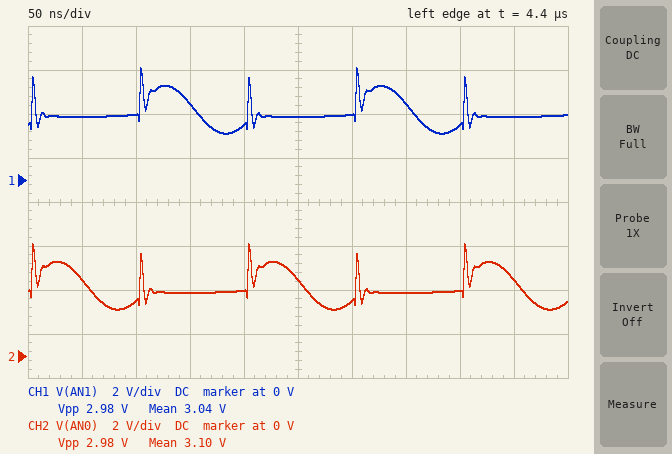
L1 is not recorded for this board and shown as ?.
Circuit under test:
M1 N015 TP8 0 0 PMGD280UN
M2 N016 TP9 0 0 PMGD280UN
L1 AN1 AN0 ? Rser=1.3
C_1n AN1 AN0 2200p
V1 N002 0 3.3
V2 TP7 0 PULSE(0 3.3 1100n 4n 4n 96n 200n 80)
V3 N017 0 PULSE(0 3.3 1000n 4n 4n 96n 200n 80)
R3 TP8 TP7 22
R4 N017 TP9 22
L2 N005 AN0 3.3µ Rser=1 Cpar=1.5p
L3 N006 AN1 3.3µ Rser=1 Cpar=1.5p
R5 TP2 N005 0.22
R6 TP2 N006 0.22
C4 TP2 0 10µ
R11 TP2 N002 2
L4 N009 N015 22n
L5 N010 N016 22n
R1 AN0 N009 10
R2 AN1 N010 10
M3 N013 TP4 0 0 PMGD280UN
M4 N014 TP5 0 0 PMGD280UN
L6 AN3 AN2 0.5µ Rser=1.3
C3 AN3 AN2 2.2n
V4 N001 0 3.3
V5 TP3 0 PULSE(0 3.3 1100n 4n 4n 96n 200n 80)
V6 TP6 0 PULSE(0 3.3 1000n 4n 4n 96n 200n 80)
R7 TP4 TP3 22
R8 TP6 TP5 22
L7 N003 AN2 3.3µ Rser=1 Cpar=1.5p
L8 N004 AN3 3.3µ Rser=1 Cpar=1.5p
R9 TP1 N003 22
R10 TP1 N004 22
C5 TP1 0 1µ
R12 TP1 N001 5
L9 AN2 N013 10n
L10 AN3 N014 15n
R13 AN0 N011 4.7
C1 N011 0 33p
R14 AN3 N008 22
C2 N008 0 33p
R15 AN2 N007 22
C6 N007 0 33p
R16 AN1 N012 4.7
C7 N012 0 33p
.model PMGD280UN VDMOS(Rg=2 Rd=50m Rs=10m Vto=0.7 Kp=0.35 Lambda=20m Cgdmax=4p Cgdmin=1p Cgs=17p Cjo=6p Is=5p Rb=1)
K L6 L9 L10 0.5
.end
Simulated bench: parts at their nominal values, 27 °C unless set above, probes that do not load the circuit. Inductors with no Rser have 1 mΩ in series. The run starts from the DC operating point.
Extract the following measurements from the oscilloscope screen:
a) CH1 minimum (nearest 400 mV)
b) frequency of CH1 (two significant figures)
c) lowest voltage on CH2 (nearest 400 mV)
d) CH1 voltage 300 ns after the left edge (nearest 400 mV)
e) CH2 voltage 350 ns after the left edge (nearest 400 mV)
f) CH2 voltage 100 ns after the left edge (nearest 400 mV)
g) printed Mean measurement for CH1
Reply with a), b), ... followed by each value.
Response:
a) 2.0 V
b) 10 MHz
c) 2.0 V
d) 2.8 V
e) 2.8 V
f) 2.4 V
g) 3.04 V
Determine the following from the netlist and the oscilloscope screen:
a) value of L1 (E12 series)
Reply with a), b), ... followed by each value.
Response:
a) 150 nH
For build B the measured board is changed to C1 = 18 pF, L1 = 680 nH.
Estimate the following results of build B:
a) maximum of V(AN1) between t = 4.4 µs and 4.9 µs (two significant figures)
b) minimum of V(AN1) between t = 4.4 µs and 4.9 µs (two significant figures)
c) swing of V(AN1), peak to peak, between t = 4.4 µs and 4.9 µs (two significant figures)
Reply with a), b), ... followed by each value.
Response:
a) 8.7 V
b) -3.4 V
c) 12 V
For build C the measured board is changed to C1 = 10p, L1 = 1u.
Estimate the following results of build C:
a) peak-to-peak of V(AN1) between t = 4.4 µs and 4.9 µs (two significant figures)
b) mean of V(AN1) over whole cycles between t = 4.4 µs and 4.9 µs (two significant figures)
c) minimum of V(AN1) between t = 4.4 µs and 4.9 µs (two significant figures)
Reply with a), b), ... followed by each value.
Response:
a) 10 V
b) 3.1 V
c) -2.3 V
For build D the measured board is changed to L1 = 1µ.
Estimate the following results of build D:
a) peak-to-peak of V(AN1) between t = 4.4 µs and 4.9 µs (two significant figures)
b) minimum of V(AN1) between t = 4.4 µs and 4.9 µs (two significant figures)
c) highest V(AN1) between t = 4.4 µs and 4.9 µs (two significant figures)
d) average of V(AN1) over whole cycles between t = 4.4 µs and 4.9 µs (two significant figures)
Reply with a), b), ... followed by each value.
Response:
a) 10 V
b) -2.4 V
c) 7.8 V
d) 3.1 V
